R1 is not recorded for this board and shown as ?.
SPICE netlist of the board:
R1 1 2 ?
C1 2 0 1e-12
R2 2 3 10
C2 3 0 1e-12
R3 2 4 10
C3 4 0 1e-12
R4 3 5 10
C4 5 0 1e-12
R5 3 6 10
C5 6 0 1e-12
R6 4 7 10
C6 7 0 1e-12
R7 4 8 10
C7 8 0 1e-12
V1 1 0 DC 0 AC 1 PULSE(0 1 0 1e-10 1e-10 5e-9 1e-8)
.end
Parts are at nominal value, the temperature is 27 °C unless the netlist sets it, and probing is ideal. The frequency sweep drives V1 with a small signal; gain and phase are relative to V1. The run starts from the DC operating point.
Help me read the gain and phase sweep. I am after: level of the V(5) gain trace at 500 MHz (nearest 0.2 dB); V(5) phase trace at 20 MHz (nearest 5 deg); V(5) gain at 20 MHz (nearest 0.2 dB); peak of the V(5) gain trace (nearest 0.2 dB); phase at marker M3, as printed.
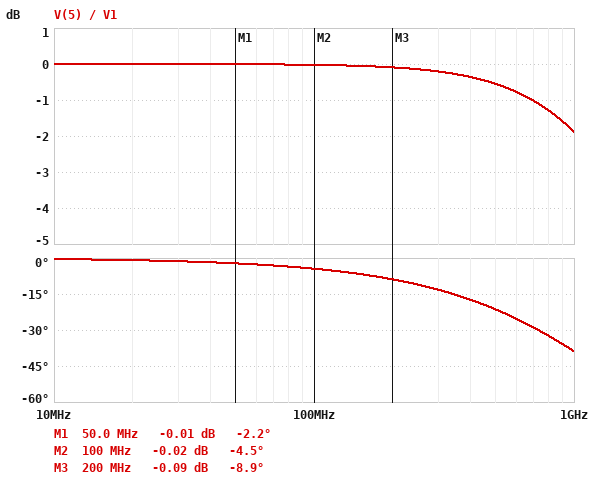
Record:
-0.6 dB
0 deg
0 dB
0 dB
-8.9 deg
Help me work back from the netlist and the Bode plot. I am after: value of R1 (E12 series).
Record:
12 Ω
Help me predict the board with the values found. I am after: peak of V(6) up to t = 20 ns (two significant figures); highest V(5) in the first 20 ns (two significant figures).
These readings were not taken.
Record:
1.0 V
1.0 V
